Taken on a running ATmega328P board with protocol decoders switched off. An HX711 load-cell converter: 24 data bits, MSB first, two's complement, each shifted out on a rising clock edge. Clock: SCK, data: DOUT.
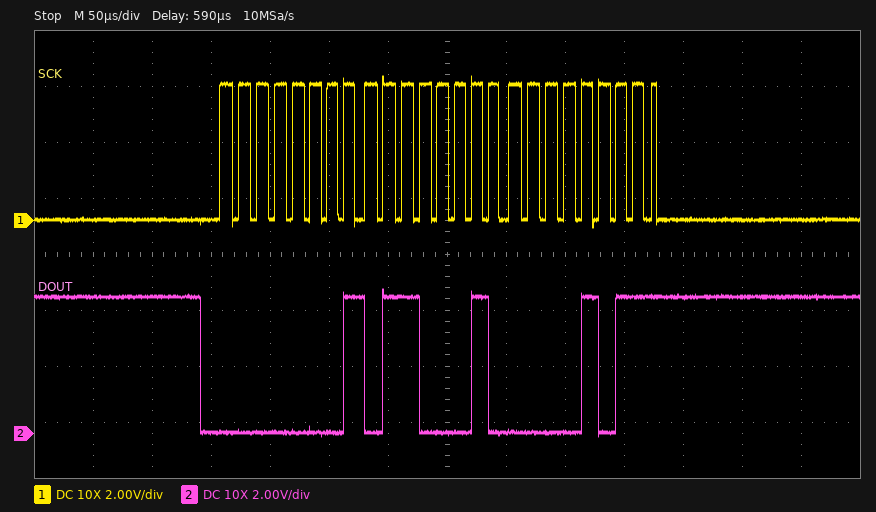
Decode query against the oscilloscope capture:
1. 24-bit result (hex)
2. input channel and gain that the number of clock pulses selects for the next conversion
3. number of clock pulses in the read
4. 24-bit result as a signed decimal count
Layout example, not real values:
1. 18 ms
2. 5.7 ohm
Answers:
1. 0x01620B
2. channel A, gain 128
3. 25
4. 90635
